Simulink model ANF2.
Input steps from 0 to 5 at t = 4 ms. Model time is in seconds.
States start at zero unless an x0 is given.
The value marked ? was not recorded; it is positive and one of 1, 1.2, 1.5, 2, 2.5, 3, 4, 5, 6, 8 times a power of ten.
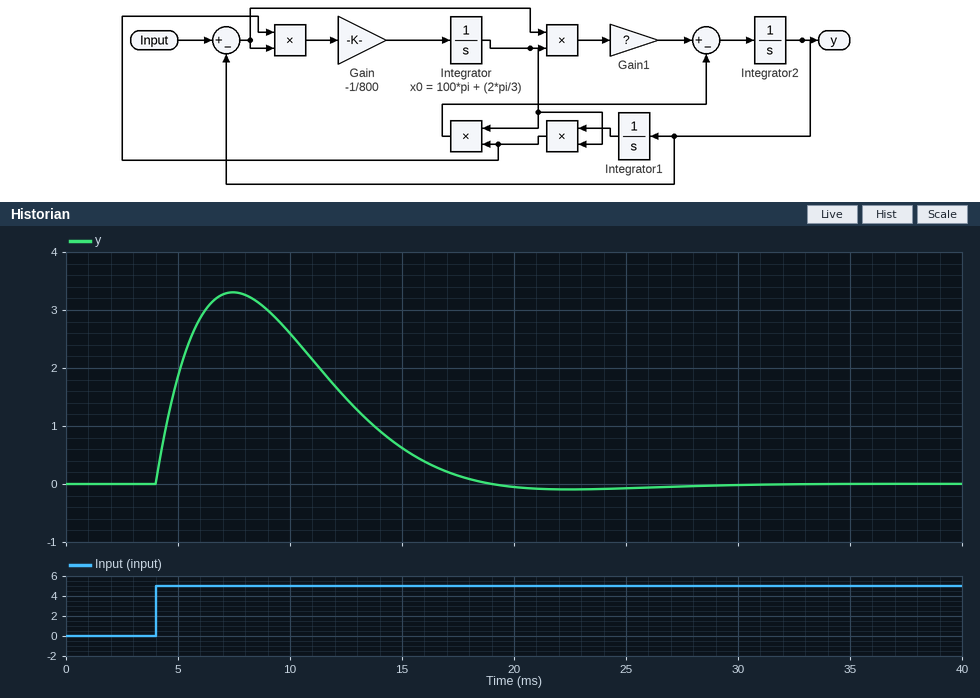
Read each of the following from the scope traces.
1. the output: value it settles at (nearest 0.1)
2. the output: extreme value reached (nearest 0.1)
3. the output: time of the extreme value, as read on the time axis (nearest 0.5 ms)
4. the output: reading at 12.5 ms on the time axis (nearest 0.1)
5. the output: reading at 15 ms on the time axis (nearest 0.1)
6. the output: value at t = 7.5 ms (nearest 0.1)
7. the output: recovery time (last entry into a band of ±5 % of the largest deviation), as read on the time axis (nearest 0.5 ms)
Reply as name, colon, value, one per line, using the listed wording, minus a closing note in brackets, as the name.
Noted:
the output: value it settles at: 0.0
the output: extreme value reached: 3.3
the output: time of the extreme value, as read on the time axis: 7.5 ms
the output: reading at 12.5 ms on the time axis: 1.5
the output: reading at 15 ms on the time axis: 0.6
the output: value at t = 7.5 ms: 3.3
the output: recovery time (last entry into a band of ±5 % of the largest deviation), as read on the time axis: 17.5 ms
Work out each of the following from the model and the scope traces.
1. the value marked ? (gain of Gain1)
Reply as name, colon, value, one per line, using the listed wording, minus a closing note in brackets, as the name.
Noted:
the value marked ?: 1.5
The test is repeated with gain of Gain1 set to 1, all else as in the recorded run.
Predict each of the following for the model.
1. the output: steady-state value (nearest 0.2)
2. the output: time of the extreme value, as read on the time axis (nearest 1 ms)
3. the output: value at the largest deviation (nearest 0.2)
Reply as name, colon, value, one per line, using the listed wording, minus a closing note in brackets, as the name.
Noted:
the output: steady-state value: 0.0
the output: time of the extreme value, as read on the time axis: 8 ms
the output: value at the largest deviation: 2.8
